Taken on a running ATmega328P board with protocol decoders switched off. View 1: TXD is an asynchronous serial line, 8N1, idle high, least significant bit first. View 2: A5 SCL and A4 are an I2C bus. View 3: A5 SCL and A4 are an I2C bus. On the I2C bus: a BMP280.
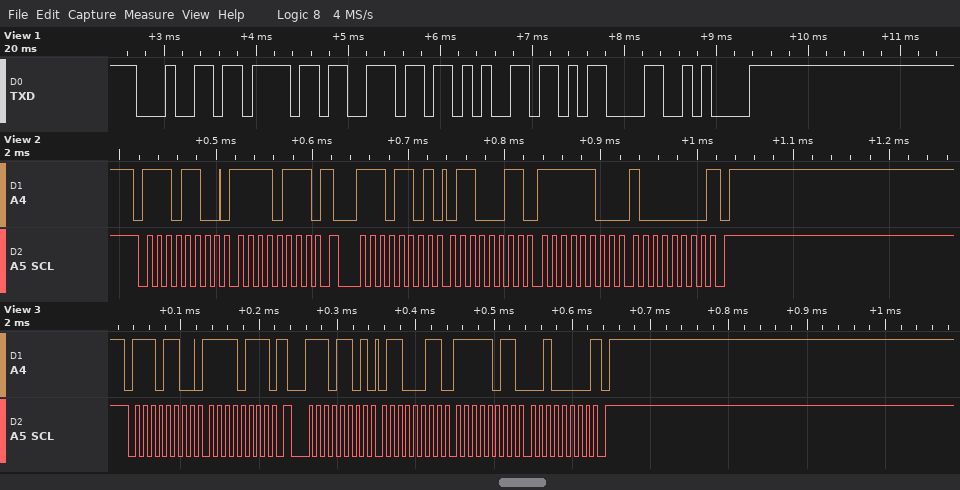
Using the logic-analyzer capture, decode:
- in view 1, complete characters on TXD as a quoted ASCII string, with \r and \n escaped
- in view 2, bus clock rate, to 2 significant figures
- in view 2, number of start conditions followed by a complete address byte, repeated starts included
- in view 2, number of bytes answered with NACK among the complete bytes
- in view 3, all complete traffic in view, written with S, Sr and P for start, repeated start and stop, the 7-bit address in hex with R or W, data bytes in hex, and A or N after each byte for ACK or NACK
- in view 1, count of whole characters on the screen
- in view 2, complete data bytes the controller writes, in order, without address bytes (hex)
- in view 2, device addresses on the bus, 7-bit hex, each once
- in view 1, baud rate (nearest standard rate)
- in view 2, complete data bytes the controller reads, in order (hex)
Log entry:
"done\r\n"
100 kHz
2
1
S 76W A F7 A Sr 76R A 63 A FB A 20 N P
6
F7
0x76
9600 baud
63 FC 80
